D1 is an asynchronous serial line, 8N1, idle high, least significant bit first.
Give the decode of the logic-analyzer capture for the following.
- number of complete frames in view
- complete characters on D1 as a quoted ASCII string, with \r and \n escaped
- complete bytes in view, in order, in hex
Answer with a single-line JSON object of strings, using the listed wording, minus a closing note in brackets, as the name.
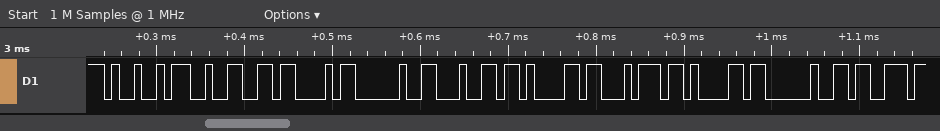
{"number of complete frames in view": "10", "complete characters on D1 as a quoted ASCII string, with \\r and \\n escaped": "\"I2C data s\"", "complete bytes in view, in order, in hex": "0x49 0x32 0x43 0x20 0x64 0x61 0x74 0x61 0x20 0x73"}
